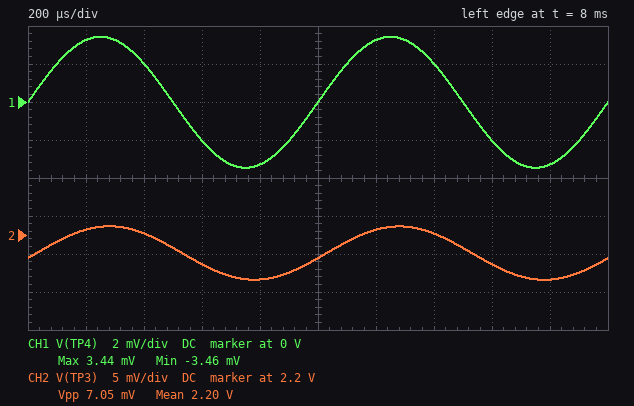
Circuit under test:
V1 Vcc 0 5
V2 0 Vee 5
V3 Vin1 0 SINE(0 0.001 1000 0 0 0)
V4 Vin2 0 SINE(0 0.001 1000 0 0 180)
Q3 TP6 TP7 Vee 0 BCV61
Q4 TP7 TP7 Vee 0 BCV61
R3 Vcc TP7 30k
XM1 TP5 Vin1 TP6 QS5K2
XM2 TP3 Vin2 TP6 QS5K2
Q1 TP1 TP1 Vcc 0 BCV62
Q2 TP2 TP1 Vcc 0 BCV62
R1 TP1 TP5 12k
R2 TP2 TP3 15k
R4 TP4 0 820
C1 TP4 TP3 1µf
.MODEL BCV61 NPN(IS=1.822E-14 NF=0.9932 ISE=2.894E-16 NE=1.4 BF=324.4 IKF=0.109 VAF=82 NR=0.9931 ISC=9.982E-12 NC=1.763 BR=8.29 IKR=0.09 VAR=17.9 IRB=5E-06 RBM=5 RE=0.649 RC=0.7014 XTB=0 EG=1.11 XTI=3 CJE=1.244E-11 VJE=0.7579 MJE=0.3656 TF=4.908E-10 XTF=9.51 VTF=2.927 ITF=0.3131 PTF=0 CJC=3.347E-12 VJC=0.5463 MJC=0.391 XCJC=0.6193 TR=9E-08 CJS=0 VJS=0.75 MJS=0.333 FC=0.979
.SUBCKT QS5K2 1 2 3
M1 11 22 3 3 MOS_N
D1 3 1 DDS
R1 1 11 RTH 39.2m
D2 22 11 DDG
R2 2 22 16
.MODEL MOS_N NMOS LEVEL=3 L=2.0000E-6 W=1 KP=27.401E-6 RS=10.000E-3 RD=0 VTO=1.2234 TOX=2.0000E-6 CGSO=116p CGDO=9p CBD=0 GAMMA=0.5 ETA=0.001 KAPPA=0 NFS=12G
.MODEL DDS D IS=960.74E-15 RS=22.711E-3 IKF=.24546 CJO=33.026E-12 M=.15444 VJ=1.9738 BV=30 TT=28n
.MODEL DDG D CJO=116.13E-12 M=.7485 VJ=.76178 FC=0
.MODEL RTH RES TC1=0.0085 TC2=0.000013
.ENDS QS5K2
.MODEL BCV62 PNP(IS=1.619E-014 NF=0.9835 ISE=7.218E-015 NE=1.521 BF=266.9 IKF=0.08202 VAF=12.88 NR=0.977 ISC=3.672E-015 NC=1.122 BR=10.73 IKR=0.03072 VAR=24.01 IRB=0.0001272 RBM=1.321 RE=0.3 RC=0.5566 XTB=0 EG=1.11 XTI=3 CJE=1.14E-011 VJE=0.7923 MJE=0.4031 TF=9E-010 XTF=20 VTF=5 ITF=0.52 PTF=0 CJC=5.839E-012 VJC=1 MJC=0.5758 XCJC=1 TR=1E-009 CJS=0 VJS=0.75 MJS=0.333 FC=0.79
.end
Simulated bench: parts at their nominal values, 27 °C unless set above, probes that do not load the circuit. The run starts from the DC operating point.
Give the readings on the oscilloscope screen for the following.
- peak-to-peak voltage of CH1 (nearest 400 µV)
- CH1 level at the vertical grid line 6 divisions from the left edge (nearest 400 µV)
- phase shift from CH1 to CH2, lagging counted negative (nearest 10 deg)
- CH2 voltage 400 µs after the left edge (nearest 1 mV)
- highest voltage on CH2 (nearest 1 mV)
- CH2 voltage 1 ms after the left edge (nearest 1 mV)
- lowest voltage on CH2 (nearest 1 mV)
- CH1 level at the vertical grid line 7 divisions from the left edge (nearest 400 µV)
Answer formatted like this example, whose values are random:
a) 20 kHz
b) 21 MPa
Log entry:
a) 6.8 mV
b) 3.2 mV
c) -10 deg
d) 2.200 V
e) 2.201 V
f) 2.197 V
g) 2.194 V
h) 2.0 mV
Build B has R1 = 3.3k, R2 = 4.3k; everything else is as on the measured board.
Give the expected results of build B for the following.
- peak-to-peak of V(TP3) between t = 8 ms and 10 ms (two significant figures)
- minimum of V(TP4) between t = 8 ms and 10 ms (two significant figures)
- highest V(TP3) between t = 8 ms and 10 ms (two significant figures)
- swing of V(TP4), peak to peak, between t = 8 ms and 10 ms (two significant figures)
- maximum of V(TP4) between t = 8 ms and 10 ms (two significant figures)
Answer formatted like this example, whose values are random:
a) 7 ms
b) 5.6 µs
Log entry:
a) 8.0 mV
b) -3.9 mV
c) 3.8 V
d) 7.8 mV
e) 3.9 mV
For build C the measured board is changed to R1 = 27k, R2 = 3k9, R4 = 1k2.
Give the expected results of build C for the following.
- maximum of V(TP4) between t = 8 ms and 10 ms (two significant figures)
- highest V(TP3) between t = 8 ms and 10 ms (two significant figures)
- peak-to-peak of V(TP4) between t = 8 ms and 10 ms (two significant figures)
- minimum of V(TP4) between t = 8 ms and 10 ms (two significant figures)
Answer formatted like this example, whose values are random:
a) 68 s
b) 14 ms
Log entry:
a) 5.2 mV
b) 1.8 V
c) 10 mV
d) -5.2 mV
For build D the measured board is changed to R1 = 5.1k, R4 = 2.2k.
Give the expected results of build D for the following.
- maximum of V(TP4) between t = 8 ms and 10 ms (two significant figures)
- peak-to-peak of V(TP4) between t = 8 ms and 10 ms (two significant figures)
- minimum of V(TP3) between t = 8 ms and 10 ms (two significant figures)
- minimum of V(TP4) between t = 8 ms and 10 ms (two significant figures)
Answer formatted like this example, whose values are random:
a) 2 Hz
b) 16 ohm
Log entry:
a) 5.5 mV
b) 11 mV
c) 2.6 V
d) -5.8 mV
